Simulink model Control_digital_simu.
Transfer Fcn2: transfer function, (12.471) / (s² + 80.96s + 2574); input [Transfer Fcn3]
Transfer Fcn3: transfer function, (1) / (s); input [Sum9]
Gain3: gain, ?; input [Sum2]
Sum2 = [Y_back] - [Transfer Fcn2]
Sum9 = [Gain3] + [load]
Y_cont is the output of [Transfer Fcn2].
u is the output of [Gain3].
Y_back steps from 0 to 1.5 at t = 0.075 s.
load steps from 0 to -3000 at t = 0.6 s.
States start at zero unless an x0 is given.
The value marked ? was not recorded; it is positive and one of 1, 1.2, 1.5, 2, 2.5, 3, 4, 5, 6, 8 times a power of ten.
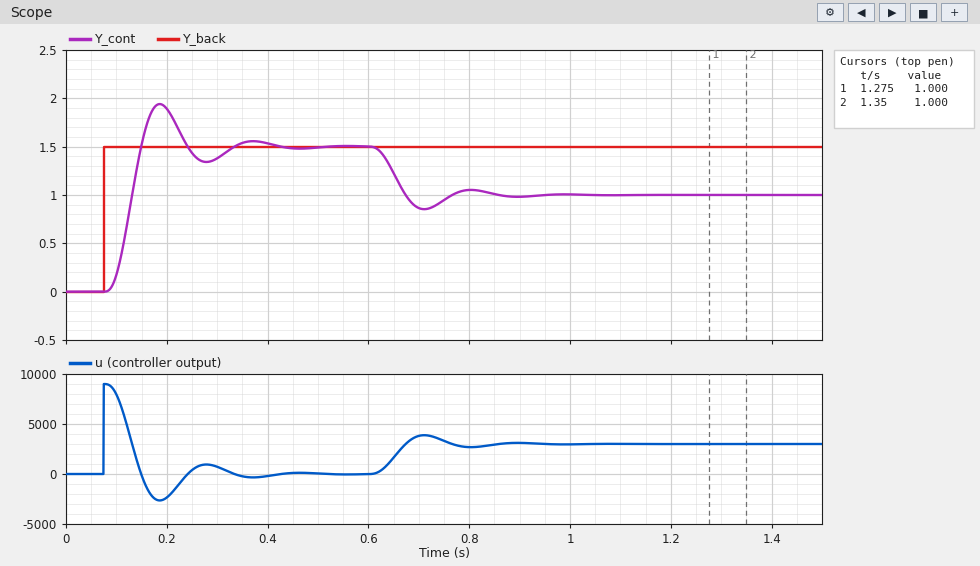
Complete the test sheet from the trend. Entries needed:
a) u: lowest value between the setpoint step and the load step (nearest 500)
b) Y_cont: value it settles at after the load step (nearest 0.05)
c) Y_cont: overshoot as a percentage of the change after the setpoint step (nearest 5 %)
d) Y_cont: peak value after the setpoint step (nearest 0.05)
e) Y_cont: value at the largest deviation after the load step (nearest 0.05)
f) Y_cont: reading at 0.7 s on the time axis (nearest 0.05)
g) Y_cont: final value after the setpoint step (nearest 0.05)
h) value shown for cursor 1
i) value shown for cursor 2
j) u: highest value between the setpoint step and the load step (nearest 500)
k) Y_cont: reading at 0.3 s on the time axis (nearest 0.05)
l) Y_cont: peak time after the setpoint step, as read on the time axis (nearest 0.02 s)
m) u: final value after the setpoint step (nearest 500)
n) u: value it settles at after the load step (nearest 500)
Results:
-2500
1.00
30 %
1.95
0.85
0.85
1.50
1.000
1.000
9000
1.40
0.18 s
0
3000
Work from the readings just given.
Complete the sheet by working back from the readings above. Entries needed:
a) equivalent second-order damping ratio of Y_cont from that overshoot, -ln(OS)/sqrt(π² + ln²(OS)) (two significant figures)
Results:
0.36
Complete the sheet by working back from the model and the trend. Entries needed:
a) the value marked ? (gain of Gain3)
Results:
6000
